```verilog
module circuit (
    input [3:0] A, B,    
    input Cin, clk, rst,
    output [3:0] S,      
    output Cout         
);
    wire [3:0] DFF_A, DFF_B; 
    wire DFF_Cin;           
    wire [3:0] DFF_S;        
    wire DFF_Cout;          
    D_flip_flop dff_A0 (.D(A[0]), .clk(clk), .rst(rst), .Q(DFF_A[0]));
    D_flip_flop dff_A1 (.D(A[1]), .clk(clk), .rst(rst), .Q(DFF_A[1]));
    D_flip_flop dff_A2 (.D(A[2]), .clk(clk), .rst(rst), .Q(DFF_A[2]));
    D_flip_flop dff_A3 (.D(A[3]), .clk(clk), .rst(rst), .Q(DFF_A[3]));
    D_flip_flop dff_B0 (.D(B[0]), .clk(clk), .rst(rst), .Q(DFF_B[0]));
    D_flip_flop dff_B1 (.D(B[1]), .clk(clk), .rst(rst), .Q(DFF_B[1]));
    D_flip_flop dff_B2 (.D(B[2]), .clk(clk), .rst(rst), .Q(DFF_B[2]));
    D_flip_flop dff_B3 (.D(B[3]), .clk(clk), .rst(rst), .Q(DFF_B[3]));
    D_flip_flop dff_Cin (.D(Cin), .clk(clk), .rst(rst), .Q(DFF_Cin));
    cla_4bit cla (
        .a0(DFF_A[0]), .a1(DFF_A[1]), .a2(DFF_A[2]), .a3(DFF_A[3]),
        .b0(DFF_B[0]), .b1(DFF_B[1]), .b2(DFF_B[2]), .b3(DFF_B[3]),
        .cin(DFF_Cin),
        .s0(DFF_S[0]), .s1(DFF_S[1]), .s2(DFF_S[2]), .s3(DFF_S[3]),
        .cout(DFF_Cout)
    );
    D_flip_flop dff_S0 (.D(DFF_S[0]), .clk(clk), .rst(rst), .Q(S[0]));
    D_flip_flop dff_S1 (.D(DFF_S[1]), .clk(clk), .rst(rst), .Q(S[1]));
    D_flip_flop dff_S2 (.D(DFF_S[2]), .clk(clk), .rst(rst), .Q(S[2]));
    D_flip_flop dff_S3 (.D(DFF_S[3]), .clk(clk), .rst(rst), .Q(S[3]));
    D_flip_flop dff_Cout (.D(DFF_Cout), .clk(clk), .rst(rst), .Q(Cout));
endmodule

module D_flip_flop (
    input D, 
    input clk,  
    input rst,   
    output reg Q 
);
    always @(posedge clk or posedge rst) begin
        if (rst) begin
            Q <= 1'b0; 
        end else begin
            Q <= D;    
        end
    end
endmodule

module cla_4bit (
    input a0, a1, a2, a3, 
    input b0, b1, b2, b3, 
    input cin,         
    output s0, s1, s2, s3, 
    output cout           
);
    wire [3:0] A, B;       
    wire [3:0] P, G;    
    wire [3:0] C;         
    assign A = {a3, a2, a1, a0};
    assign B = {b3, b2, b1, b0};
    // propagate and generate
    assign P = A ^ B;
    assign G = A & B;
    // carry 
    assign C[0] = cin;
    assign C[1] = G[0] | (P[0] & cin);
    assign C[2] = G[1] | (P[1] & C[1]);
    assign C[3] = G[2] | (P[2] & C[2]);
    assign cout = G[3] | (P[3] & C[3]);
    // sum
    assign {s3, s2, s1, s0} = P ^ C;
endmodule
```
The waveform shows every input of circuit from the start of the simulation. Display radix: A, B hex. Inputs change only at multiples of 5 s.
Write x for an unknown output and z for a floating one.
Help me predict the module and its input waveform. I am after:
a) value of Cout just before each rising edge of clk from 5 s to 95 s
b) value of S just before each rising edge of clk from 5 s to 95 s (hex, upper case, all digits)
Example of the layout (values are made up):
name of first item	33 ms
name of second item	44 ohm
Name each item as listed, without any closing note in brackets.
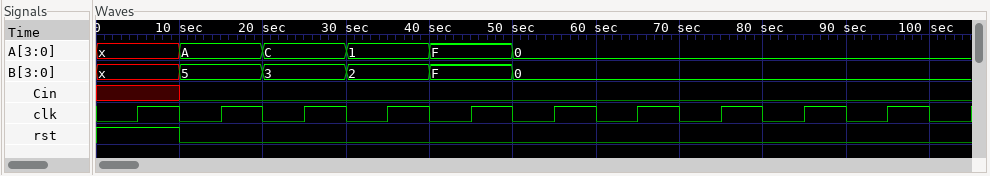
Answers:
value of Cout just before each rising edge of clk from 5 s to 95 s	0 0 0 0 0 0 1 0 0 0
value of S just before each rising edge of clk from 5 s to 95 s	0, 0, 0, F, F, 3, E, 0, 0, 0
